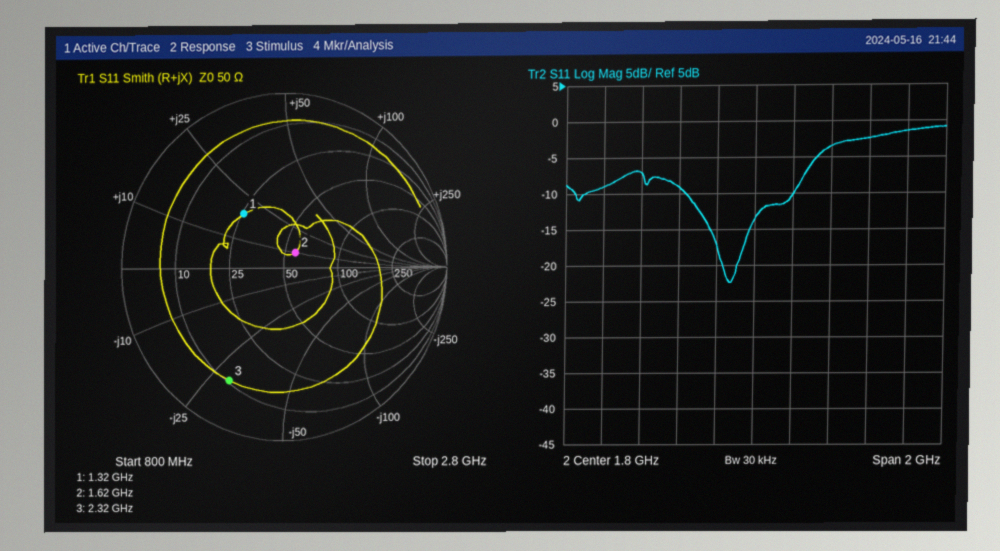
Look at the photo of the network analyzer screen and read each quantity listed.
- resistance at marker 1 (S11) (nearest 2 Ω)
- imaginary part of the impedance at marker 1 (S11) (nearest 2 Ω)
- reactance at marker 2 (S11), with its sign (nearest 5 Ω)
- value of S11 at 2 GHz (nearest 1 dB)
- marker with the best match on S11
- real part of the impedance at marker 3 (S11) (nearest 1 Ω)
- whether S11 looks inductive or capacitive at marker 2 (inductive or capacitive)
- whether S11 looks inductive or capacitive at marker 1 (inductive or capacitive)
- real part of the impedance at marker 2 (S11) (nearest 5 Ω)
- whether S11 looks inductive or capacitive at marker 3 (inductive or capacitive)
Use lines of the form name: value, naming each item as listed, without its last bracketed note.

resistance at marker 1 (S11): 26 Ω
imaginary part of the impedance at marker 1 (S11): +18 Ω
reactance at marker 2 (S11), with its sign: +10 Ω
value of S11 at 2 GHz: -10 dB
marker with the best match on S11: marker 2
real part of the impedance at marker 3 (S11): 11 Ω
whether S11 looks inductive or capacitive at marker 2: inductive
whether S11 looks inductive or capacitive at marker 1: inductive
real part of the impedance at marker 2 (S11): 55 Ω
whether S11 looks inductive or capacitive at marker 3: capacitive
